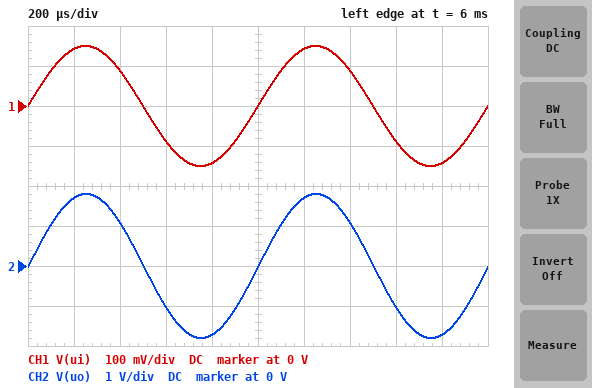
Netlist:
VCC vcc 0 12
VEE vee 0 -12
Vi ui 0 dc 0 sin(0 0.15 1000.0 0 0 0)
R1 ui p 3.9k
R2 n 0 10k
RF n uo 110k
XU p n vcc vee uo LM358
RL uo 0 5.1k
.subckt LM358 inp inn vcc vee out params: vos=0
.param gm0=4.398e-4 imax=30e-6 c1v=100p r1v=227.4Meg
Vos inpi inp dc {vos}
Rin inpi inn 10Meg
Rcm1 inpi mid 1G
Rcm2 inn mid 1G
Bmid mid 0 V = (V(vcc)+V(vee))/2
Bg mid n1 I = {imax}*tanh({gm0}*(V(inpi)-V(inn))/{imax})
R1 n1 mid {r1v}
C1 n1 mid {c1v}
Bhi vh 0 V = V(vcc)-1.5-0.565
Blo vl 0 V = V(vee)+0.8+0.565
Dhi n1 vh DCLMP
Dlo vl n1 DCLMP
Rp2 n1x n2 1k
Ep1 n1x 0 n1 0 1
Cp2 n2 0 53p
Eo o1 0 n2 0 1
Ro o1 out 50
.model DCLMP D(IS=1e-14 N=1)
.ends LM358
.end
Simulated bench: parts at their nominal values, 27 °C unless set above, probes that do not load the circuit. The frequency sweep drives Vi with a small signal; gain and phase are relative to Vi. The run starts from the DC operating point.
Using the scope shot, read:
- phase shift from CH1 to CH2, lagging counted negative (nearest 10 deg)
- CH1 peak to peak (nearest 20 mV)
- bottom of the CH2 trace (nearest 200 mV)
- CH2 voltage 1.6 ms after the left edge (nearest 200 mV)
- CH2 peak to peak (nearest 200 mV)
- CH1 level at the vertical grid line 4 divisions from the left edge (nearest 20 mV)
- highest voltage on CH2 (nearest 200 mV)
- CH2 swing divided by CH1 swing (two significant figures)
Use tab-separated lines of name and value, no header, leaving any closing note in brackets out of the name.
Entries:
phase shift from CH1 to CH2, lagging counted negative	0 deg
CH1 peak to peak	300 mV
bottom of the CH2 trace	-1.8 V
CH2 voltage 1.6 ms after the left edge	-1.0 V
CH2 peak to peak	3.6 V
CH1 level at the vertical grid line 4 divisions from the left edge	-140 mV
highest voltage on CH2	1.8 V
CH2 swing divided by CH1 swing	12
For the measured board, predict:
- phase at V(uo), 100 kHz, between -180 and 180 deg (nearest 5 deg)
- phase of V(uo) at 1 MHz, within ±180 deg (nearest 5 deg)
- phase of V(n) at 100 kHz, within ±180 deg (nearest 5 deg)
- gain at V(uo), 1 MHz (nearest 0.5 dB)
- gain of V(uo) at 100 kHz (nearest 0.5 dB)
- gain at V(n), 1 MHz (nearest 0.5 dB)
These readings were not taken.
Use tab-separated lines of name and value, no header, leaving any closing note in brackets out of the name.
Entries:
phase at V(uo), 100 kHz, between -180 and 180 deg	-60 deg
phase of V(uo) at 1 MHz, within ±180 deg	-105 deg
phase of V(n) at 100 kHz, within ±180 deg	-60 deg
gain at V(uo), 1 MHz	-3.5 dB
gain of V(uo) at 100 kHz	15.5 dB
gain at V(n), 1 MHz	-25.0 dB
